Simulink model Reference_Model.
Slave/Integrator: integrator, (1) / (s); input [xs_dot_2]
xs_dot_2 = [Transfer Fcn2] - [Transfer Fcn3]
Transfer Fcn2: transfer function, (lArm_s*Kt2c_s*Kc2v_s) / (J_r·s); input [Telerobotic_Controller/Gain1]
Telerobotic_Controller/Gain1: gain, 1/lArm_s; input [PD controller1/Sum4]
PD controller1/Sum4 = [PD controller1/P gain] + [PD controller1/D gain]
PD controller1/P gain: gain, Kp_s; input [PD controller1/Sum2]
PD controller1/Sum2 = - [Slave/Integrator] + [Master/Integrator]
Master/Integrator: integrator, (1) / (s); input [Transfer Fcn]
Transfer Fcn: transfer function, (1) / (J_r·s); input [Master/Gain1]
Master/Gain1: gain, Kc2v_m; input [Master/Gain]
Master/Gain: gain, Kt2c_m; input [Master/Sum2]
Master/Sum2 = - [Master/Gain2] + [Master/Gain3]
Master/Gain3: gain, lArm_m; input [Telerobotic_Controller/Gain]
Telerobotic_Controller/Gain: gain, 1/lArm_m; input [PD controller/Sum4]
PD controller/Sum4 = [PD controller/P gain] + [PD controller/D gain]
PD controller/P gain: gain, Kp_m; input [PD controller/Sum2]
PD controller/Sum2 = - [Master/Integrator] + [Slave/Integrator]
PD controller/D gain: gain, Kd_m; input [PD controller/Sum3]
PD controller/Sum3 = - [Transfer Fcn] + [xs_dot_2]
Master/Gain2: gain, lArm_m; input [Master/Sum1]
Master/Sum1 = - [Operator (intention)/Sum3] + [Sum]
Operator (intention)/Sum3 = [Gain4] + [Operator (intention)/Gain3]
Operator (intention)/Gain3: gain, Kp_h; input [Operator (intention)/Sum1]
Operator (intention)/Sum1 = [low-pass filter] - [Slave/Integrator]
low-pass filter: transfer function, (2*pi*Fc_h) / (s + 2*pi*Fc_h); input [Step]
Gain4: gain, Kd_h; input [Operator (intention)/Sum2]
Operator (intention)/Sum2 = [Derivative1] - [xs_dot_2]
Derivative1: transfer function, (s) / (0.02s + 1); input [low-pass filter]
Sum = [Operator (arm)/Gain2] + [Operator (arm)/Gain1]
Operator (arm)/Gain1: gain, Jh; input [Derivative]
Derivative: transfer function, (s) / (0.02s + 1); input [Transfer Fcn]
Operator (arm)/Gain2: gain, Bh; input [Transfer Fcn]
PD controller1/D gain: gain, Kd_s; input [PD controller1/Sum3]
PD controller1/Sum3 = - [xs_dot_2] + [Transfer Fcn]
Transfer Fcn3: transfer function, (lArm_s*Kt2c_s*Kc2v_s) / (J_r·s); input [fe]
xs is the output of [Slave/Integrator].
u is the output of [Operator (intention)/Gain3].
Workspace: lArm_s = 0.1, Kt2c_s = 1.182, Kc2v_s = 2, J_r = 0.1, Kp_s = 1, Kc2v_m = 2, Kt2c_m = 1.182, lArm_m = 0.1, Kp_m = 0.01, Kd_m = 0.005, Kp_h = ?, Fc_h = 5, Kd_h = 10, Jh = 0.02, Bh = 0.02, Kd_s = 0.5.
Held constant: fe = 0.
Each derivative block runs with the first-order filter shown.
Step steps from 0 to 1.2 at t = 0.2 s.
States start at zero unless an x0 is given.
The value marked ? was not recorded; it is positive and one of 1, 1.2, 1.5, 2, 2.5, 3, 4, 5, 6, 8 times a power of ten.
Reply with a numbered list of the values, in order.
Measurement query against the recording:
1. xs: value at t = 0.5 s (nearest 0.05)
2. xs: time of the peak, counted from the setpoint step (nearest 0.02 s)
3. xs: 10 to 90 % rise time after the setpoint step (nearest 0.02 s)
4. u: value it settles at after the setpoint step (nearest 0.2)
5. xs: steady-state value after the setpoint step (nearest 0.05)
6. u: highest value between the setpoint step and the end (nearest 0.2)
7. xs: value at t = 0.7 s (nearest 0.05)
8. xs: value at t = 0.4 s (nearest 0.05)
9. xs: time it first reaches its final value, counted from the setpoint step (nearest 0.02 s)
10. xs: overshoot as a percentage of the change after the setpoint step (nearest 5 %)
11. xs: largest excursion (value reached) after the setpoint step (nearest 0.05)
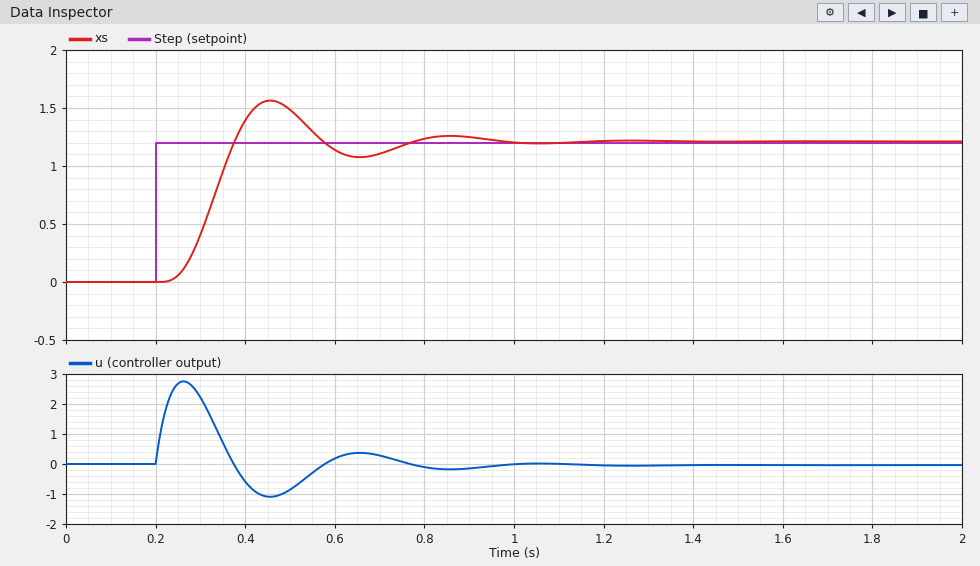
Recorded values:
1. 1.50
2. 0.26 s
3. 0.10 s
4. 0.0
5. 1.20
6. 2.8
7. 1.10
8. 1.40
9. 0.18 s
10. 30 %
11. 1.55
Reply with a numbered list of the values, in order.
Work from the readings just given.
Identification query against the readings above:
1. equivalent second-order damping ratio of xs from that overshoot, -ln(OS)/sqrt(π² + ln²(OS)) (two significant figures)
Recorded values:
1. 0.36
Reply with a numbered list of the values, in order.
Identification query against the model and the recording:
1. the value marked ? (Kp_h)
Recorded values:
1. 3
